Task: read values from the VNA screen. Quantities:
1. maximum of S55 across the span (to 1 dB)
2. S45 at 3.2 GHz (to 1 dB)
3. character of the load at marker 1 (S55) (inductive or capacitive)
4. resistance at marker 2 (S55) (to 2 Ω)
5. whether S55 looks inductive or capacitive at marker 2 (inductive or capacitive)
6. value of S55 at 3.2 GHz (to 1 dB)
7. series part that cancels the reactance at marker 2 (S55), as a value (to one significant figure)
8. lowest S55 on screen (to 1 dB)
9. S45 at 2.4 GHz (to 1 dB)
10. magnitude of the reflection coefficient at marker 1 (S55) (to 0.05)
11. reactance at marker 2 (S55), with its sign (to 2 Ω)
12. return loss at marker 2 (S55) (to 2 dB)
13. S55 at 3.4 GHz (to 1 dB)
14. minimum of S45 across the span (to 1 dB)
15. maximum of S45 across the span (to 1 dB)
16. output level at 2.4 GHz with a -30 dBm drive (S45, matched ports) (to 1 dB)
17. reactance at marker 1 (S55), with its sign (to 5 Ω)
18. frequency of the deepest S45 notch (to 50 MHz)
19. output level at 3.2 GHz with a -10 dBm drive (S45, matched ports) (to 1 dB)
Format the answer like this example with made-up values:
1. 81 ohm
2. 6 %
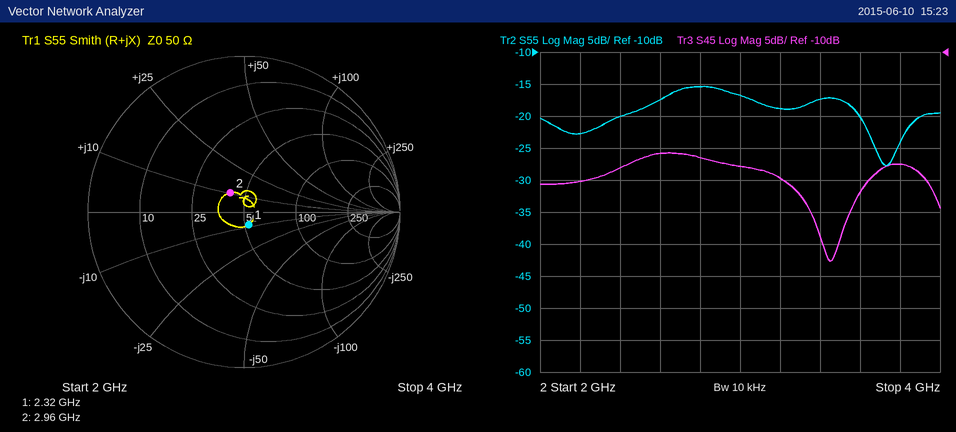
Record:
1. -15 dB
2. -30 dB
3. capacitive
4. 40 Ω
5. inductive
6. -19 dB
7. 5 pF
8. -28 dB
9. -28 dB
10. 0.10
11. +10 Ω
12. 16 dB
13. -17 dB
14. -43 dB
15. -26 dB
16. -58 dBm
17. -10 Ω
18. 3.45 GHz
19. -40 dBm
